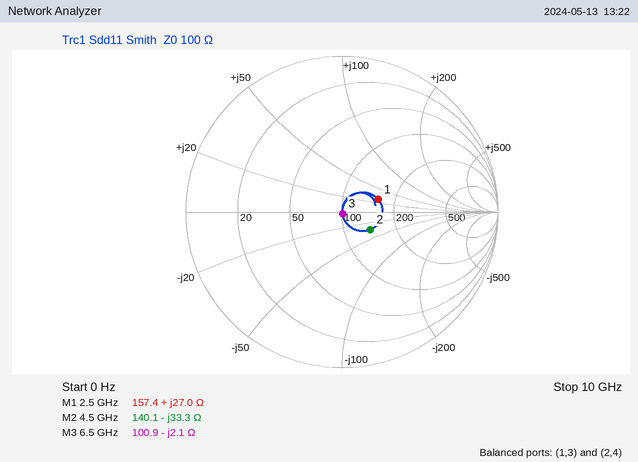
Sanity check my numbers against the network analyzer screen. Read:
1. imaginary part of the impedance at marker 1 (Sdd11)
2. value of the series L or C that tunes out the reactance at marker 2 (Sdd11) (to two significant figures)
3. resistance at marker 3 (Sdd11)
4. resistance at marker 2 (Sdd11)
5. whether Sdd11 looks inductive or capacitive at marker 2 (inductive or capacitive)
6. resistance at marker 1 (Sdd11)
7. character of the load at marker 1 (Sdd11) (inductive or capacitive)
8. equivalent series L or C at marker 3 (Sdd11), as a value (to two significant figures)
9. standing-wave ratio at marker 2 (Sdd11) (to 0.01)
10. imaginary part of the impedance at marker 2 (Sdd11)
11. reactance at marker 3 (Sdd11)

+27.0 Ω
1.2 nH
100.9 Ω
140.1 Ω
capacitive
157.4 Ω
inductive
12 pF
1.55
-33.3 Ω
-2.1 Ω
